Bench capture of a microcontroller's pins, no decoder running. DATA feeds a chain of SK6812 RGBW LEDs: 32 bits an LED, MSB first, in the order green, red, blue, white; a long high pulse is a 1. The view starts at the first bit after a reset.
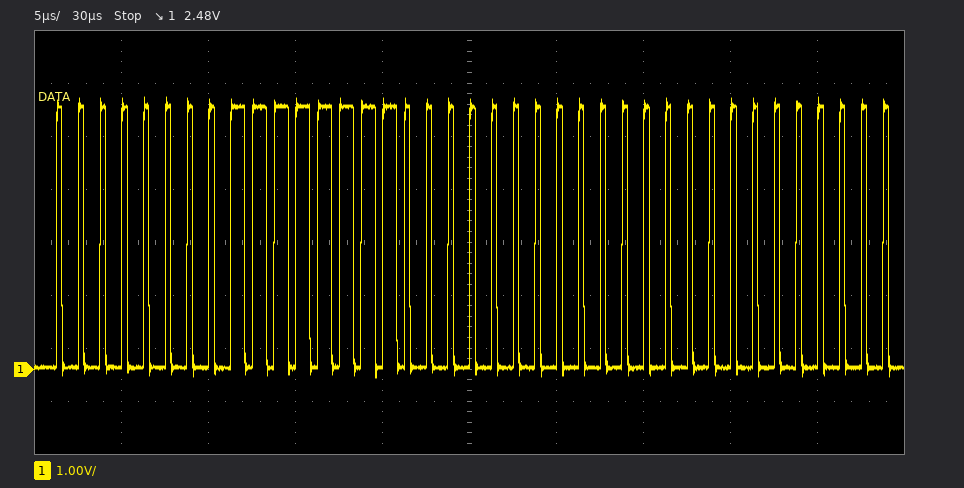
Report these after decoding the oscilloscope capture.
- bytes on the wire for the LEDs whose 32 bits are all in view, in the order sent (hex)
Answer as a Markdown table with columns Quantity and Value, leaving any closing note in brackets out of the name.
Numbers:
| Quantity | Value |
|---|---|
| bytes on the wire for the LEDs whose 32 bits are all in view, in the order sent | 00 FF 00 00 |
